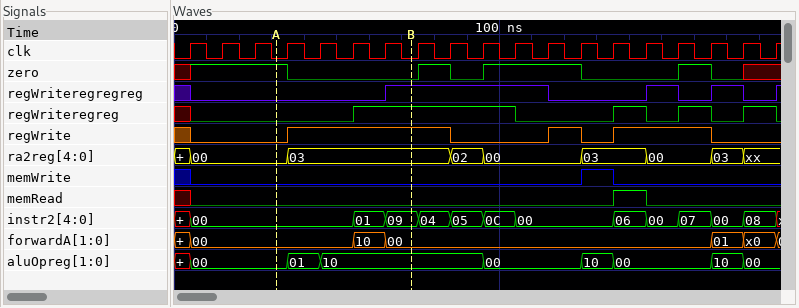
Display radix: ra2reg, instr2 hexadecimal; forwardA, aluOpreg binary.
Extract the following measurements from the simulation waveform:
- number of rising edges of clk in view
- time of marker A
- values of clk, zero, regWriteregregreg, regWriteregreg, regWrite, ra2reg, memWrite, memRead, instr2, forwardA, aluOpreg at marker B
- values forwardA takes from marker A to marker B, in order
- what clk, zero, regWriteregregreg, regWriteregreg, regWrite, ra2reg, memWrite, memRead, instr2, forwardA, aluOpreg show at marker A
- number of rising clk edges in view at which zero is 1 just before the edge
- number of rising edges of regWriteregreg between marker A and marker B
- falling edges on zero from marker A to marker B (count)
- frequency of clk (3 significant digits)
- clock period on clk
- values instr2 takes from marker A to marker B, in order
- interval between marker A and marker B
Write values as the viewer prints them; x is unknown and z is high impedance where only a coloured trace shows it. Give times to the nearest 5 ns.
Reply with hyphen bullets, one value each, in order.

- 19
- 30 ns
- clk=0, zero=0, regWriteregregreg=1, regWriteregreg=1, regWrite=1, ra2reg=03, memWrite=0, memRead=0, instr2=09, forwardA=00, aluOpreg=10
- 00, 10, 00
- clk=0, zero=1, regWriteregregreg=0, regWriteregreg=0, regWrite=0, ra2reg=00, memWrite=0, memRead=0, instr2=00, forwardA=00, aluOpreg=00
- 8
- 1
- 1
- 100 MHz
- 10 ns
- 00, 01, 09
- 40 ns
